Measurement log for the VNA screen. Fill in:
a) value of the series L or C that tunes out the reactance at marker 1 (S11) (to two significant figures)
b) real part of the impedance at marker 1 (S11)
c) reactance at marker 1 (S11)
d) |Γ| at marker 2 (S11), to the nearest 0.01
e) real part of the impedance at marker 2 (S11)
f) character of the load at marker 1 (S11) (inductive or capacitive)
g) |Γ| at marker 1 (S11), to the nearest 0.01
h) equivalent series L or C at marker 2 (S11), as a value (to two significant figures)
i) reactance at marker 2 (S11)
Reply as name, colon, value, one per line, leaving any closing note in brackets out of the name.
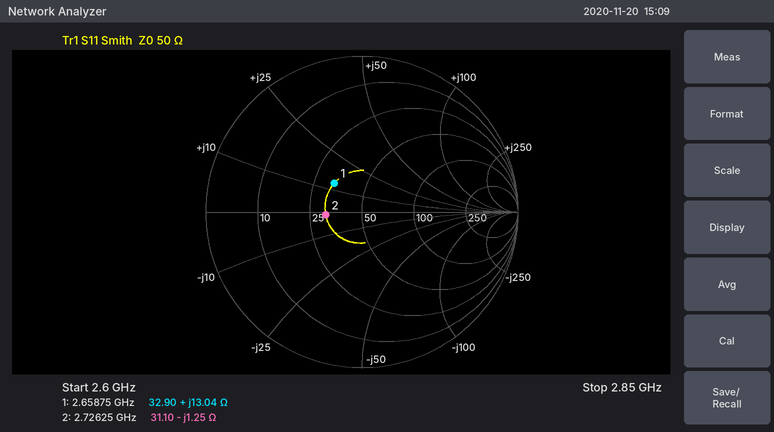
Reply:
value of the series L or C that tunes out the reactance at marker 1 (S11): 4.6 pF
real part of the impedance at marker 1: 32.90 Ω
reactance at marker 1: +13.04 Ω
|Γ| at marker 2 (S11), to the nearest 0.01: 0.23
real part of the impedance at marker 2: 31.10 Ω
character of the load at marker 1 (S11): inductive
|Γ| at marker 1 (S11), to the nearest 0.01: 0.26
equivalent series L or C at marker 2 (S11), as a value: 47 pF
reactance at marker 2: -1.25 Ω
